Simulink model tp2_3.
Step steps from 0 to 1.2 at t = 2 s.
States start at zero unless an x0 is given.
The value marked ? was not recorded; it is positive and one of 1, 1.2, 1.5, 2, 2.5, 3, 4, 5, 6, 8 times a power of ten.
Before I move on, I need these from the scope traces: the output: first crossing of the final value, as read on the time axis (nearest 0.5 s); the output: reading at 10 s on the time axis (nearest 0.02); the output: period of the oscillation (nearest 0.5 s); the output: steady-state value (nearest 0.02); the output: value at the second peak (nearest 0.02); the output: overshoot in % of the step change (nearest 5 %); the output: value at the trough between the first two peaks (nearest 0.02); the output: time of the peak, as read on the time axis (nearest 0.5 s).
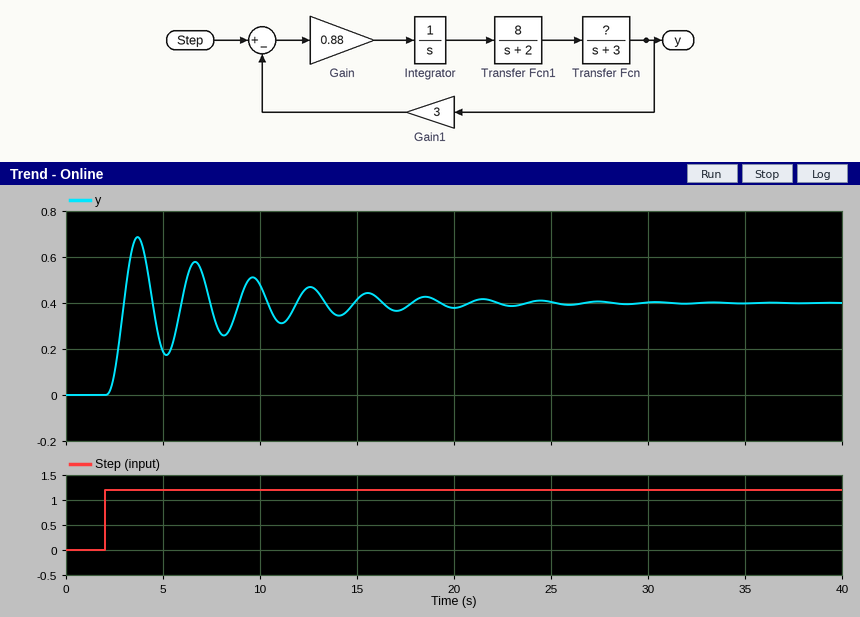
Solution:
3.0 s
0.48
3.0 s
0.40
0.58
70 %
0.18
3.5 s
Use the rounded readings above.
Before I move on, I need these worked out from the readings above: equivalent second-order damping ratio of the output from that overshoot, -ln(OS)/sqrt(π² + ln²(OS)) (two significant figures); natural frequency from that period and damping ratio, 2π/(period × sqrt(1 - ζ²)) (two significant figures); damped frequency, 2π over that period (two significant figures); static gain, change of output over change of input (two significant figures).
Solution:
0.11
2.1 rad/s
2.1 rad/s
0.33
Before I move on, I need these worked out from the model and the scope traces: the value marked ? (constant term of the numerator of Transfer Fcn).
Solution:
1
